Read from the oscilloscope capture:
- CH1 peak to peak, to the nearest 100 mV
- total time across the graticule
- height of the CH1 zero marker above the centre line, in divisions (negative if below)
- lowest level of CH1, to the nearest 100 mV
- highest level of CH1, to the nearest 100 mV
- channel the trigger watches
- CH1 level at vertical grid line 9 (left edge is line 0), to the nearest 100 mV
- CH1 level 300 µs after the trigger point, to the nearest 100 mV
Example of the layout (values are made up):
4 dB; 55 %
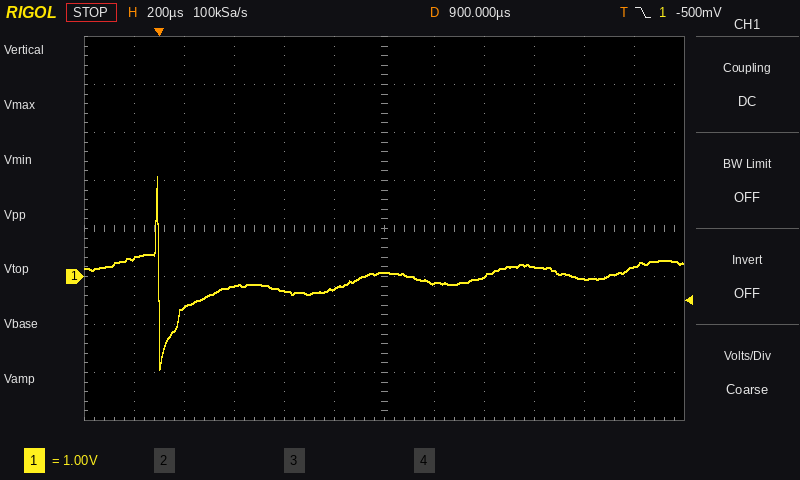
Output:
4.0 V; 2.4 ms; -1.0 div; -1.9 V; 2.1 V; CH1; 200 mV; -200 mV
